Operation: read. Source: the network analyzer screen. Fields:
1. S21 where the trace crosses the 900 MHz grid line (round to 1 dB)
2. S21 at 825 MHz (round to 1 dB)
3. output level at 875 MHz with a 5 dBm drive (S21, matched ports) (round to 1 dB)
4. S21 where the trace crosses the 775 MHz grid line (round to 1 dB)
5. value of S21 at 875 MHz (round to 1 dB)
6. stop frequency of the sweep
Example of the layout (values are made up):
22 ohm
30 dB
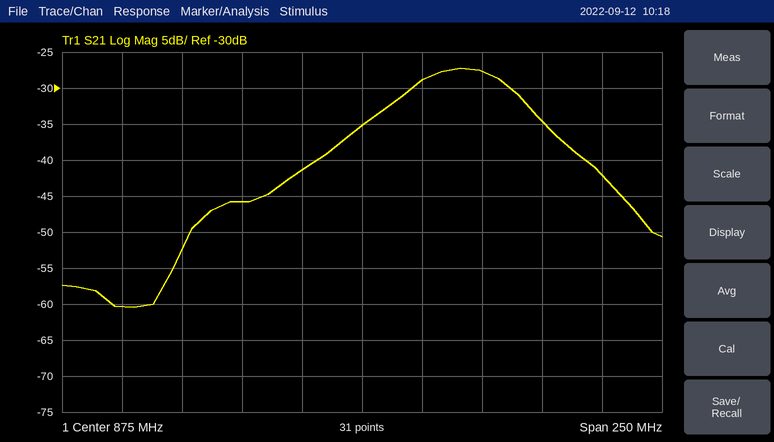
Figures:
-29 dB
-46 dB
-30 dBm
-60 dB
-35 dB
1 GHz
